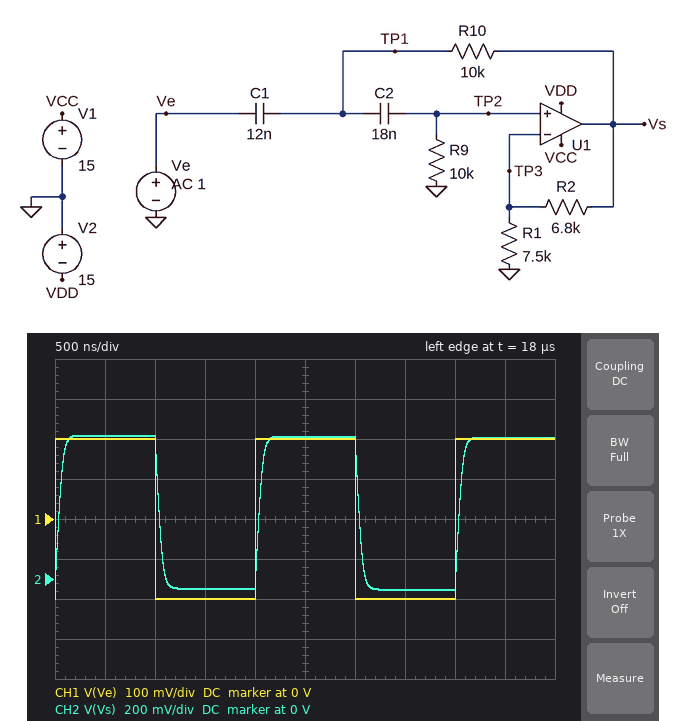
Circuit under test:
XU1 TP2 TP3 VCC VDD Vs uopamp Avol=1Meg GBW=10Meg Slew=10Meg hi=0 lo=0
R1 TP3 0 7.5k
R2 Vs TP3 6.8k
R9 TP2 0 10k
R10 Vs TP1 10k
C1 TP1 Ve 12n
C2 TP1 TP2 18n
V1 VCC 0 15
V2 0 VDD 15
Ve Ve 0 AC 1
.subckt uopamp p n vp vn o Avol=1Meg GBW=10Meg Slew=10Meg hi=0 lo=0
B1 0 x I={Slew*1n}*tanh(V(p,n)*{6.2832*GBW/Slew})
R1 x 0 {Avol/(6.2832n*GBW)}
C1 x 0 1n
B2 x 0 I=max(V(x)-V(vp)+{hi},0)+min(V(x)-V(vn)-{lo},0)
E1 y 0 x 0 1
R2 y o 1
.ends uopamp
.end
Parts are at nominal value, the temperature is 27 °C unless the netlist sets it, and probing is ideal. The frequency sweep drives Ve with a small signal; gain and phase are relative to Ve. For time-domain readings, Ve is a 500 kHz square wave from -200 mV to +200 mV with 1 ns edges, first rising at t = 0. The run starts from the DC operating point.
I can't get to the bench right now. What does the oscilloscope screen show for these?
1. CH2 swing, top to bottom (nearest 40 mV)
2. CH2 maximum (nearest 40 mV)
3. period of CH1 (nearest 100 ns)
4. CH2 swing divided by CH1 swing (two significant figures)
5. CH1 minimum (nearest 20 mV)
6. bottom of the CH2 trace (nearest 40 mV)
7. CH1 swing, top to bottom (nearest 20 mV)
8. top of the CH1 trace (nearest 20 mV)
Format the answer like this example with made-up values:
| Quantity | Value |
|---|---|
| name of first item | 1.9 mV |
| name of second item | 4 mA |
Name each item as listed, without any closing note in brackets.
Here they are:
| Quantity | Value |
|---|---|
| CH2 swing, top to bottom | 760 mV |
| CH2 maximum | 720 mV |
| period of CH1 | 2.0 µs |
| CH2 swing divided by CH1 swing | 1.9 |
| CH1 minimum | -200 mV |
| bottom of the CH2 trace | -40 mV |
| CH1 swing, top to bottom | 400 mV |
| top of the CH1 trace | 200 mV |
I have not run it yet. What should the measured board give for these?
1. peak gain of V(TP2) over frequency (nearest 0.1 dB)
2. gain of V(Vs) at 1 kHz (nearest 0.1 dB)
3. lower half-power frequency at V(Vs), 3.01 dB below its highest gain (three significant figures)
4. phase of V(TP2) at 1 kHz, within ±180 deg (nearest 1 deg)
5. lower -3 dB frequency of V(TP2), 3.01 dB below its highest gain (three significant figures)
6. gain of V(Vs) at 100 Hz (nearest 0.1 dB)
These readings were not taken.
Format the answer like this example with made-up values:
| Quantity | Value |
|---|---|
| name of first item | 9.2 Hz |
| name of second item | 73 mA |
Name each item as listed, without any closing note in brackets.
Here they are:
| Quantity | Value |
|---|---|
| peak gain of V(TP2) over frequency | 1.7 dB |
| gain of V(Vs) at 1 kHz | 5.4 dB |
| lower half-power frequency at V(Vs), 3.01 dB below its highest gain | 918 Hz |
| phase of V(TP2) at 1 kHz, within ±180 deg | 100 deg |
| lower -3 dB frequency of V(TP2), 3.01 dB below its highest gain | 918 Hz |
| gain of V(Vs) at 100 Hz | -35.7 dB |
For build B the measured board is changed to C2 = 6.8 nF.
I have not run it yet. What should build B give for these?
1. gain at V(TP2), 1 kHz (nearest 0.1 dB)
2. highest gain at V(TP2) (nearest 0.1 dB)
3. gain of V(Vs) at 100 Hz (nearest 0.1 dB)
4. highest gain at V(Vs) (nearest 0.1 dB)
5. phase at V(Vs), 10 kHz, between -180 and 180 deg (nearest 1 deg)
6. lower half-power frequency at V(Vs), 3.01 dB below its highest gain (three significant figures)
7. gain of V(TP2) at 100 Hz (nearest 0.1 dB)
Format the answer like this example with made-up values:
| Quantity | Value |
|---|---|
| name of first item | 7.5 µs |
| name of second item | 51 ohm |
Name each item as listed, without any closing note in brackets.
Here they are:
| Quantity | Value |
|---|---|
| gain at V(TP2), 1 kHz | -10.2 dB |
| highest gain at V(TP2) | 0 dB |
| gain of V(Vs) at 100 Hz | -44.2 dB |
| highest gain at V(Vs) | 5.6 dB |
| phase at V(Vs), 10 kHz, between -180 and 180 deg | 14 deg |
| lower half-power frequency at V(Vs), 3.01 dB below its highest gain | 1.74 kHz |
| gain of V(TP2) at 100 Hz | -49.8 dB |
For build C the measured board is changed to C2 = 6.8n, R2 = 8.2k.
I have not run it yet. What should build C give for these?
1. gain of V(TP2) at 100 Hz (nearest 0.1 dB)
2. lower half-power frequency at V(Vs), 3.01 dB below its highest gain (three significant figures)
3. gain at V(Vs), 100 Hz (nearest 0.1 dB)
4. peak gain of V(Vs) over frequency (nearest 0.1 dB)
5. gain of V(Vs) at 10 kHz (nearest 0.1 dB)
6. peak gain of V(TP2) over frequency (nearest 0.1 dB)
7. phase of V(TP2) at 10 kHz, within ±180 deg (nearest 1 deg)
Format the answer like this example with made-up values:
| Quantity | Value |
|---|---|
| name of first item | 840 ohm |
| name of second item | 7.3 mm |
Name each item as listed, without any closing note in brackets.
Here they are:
| Quantity | Value |
|---|---|
| gain of V(TP2) at 100 Hz | -49.8 dB |
| lower half-power frequency at V(Vs), 3.01 dB below its highest gain | 1.62 kHz |
| gain at V(Vs), 100 Hz | -43.4 dB |
| peak gain of V(Vs) over frequency | 6.6 dB |
| gain of V(Vs) at 10 kHz | 6.5 dB |
| peak gain of V(TP2) over frequency | 0.2 dB |
| phase of V(TP2) at 10 kHz, within ±180 deg | 13 deg |
